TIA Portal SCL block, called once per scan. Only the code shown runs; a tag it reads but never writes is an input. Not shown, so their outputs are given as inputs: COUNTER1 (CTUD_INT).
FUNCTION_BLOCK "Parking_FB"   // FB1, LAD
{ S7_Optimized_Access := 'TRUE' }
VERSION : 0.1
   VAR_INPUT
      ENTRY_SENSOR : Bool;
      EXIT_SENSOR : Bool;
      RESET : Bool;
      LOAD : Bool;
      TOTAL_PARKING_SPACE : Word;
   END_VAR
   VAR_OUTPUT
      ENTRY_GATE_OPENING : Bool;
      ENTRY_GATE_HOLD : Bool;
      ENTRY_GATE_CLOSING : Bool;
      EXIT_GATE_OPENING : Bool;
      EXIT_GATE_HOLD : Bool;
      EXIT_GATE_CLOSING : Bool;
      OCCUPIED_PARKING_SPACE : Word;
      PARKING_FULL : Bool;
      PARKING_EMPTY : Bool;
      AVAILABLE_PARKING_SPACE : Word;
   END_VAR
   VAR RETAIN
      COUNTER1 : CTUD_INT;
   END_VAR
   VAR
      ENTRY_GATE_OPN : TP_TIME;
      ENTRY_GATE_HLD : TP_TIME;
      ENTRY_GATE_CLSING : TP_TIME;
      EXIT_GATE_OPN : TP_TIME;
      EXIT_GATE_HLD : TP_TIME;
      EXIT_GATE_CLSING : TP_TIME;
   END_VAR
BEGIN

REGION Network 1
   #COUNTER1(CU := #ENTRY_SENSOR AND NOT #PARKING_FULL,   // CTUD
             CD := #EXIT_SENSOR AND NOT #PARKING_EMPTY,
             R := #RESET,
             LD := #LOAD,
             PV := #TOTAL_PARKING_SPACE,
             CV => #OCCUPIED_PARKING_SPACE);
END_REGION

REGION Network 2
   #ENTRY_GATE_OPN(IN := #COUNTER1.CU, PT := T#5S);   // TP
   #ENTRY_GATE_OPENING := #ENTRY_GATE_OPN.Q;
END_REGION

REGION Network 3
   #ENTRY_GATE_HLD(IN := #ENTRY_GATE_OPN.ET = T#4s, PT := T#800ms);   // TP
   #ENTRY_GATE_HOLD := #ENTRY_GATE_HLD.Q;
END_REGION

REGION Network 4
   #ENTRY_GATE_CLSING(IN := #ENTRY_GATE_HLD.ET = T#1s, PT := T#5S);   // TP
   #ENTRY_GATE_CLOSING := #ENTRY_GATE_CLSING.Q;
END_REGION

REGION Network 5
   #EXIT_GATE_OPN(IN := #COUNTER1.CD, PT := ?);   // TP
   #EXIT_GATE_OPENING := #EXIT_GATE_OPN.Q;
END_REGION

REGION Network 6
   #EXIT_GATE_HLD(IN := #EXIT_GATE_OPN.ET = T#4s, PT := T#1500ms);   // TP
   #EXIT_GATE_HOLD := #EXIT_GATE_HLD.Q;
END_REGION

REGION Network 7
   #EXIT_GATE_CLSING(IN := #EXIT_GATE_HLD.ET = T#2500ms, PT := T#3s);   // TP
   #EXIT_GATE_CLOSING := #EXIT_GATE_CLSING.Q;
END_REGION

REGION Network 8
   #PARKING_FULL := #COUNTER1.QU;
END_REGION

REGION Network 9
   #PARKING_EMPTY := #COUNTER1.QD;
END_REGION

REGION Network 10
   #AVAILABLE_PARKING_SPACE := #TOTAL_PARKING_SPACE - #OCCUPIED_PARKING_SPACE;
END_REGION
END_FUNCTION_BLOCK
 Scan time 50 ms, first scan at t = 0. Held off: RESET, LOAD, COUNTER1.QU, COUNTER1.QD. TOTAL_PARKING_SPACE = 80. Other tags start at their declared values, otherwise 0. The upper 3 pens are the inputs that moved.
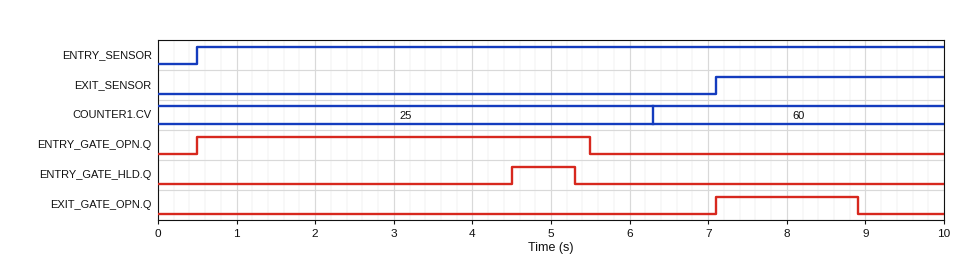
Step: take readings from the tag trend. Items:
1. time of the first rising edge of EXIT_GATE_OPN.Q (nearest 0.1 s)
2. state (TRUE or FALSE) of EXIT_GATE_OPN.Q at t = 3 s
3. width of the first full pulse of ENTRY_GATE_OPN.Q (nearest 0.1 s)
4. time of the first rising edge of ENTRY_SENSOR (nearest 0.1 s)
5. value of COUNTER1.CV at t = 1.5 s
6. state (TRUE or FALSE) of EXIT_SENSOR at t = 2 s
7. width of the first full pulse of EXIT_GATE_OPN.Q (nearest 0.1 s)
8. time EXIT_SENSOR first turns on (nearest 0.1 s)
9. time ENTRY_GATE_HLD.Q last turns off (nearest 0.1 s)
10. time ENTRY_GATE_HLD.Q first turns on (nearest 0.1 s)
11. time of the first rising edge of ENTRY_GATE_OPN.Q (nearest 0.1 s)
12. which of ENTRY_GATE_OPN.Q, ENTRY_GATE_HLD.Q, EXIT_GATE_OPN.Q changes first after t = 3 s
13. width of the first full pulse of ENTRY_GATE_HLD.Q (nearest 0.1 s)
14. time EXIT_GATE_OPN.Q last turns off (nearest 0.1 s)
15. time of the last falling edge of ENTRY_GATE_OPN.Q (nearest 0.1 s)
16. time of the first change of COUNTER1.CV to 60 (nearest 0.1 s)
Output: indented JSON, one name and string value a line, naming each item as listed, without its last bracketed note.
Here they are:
{
  "time of the first rising edge of EXIT_GATE_OPN.Q": "7.1 s",
  "state (TRUE or FALSE) of EXIT_GATE_OPN.Q at t = 3 s": "FALSE",
  "width of the first full pulse of ENTRY_GATE_OPN.Q": "5.0 s",
  "time of the first rising edge of ENTRY_SENSOR": "0.5 s",
  "value of COUNTER1.CV at t = 1.5 s": "25",
  "state (TRUE or FALSE) of EXIT_SENSOR at t = 2 s": "FALSE",
  "width of the first full pulse of EXIT_GATE_OPN.Q": "1.8 s",
  "time EXIT_SENSOR first turns on": "7.1 s",
  "time ENTRY_GATE_HLD.Q last turns off": "5.3 s",
  "time ENTRY_GATE_HLD.Q first turns on": "4.5 s",
  "time of the first rising edge of ENTRY_GATE_OPN.Q": "0.5 s",
  "which of ENTRY_GATE_OPN.Q, ENTRY_GATE_HLD.Q, EXIT_GATE_OPN.Q changes first after t = 3 s": "ENTRY_GATE_HLD.Q",
  "width of the first full pulse of ENTRY_GATE_HLD.Q": "0.8 s",
  "time EXIT_GATE_OPN.Q last turns off": "8.9 s",
  "time of the last falling edge of ENTRY_GATE_OPN.Q": "5.5 s",
  "time of the first change of COUNTER1.CV to 60": "6.3 s"
}
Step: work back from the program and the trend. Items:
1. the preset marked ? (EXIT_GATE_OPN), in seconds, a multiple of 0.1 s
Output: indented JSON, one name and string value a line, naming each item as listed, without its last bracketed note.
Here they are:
{
  "the preset marked ? (EXIT_GATE_OPN), in seconds, a multiple of 0.1 s": "1.8 s"
}
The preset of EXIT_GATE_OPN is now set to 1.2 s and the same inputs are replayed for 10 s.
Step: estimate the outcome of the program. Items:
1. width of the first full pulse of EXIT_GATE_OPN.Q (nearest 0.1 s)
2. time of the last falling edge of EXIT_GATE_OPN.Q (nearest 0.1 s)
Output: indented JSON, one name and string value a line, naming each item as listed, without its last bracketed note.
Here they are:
{
  "width of the first full pulse of EXIT_GATE_OPN.Q": "1.2 s",
  "time of the last falling edge of EXIT_GATE_OPN.Q": "8.3 s"
}
